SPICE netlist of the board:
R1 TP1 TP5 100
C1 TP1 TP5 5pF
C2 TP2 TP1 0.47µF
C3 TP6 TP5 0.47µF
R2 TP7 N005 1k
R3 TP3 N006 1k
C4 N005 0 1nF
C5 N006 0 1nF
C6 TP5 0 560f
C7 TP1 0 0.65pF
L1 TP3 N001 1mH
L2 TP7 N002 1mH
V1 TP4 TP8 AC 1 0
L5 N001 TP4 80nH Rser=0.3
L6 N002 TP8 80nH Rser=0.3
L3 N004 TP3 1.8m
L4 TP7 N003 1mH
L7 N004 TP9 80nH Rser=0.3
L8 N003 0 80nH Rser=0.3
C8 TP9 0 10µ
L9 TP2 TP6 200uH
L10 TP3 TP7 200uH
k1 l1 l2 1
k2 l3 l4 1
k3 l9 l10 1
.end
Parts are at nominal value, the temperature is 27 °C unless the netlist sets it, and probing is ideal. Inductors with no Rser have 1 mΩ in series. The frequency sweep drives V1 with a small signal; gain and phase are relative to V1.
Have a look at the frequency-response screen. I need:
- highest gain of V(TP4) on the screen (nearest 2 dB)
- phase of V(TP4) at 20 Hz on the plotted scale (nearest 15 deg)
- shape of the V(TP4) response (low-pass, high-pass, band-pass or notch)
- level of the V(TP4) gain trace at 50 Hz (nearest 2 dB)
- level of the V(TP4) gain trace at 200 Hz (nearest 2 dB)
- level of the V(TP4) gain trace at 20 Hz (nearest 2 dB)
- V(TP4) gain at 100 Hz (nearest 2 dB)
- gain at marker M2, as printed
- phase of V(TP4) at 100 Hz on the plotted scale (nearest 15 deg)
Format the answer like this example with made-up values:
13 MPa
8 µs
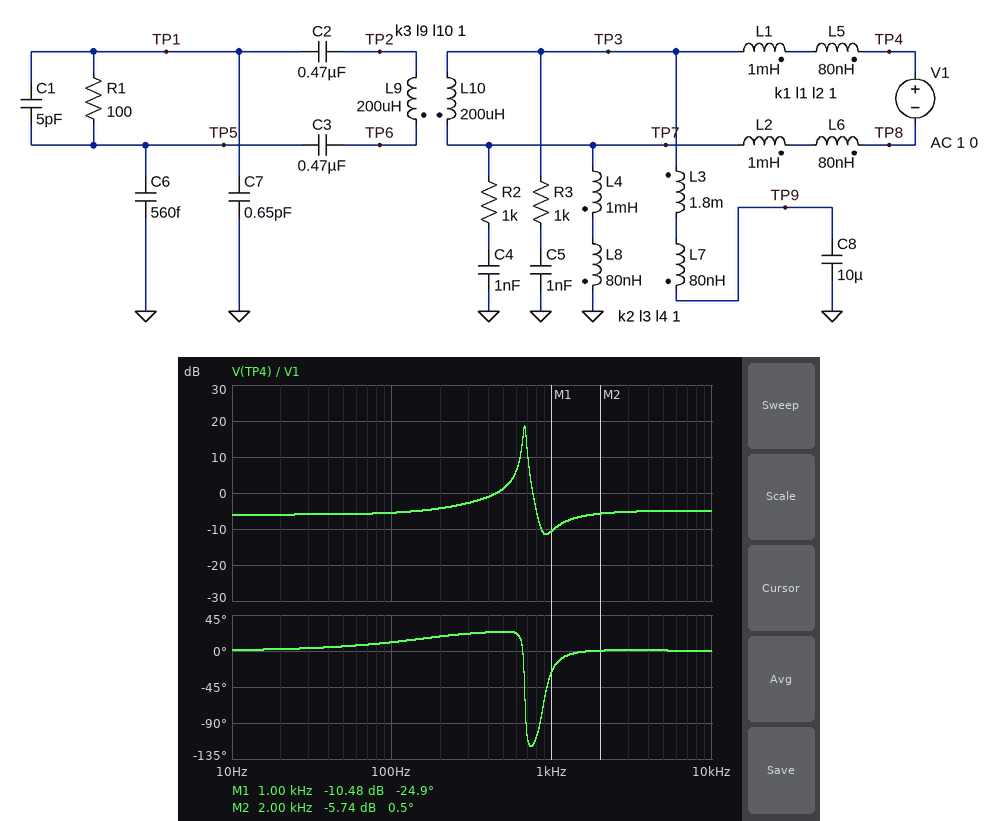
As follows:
18 dB
0 deg
band-pass
-6 dB
-4 dB
-6 dB
-6 dB
-5.74 dB
15 deg
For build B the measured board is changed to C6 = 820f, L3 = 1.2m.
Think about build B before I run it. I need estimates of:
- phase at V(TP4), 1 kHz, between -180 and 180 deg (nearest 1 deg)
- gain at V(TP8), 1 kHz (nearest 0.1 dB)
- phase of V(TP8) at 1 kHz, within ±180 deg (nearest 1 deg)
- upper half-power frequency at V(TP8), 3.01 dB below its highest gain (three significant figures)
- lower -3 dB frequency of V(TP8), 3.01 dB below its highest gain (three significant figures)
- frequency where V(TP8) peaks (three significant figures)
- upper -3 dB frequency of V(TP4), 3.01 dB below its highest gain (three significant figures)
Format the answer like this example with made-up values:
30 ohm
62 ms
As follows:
-85 deg
0.1 dB
-164 deg
775 Hz
737 Hz
755 Hz
771 Hz
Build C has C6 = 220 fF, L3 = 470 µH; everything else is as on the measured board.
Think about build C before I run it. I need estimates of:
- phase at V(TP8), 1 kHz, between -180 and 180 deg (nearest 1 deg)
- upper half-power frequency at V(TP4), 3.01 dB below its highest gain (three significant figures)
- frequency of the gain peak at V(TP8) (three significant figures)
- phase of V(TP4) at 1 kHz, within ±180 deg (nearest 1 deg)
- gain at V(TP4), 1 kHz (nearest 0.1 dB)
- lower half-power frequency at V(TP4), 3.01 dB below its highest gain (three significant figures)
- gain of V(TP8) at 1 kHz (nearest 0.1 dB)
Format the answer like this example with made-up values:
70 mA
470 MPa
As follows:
-134 deg
964 Hz
938 Hz
-121 deg
10.3 dB
903 Hz
11.8 dB
